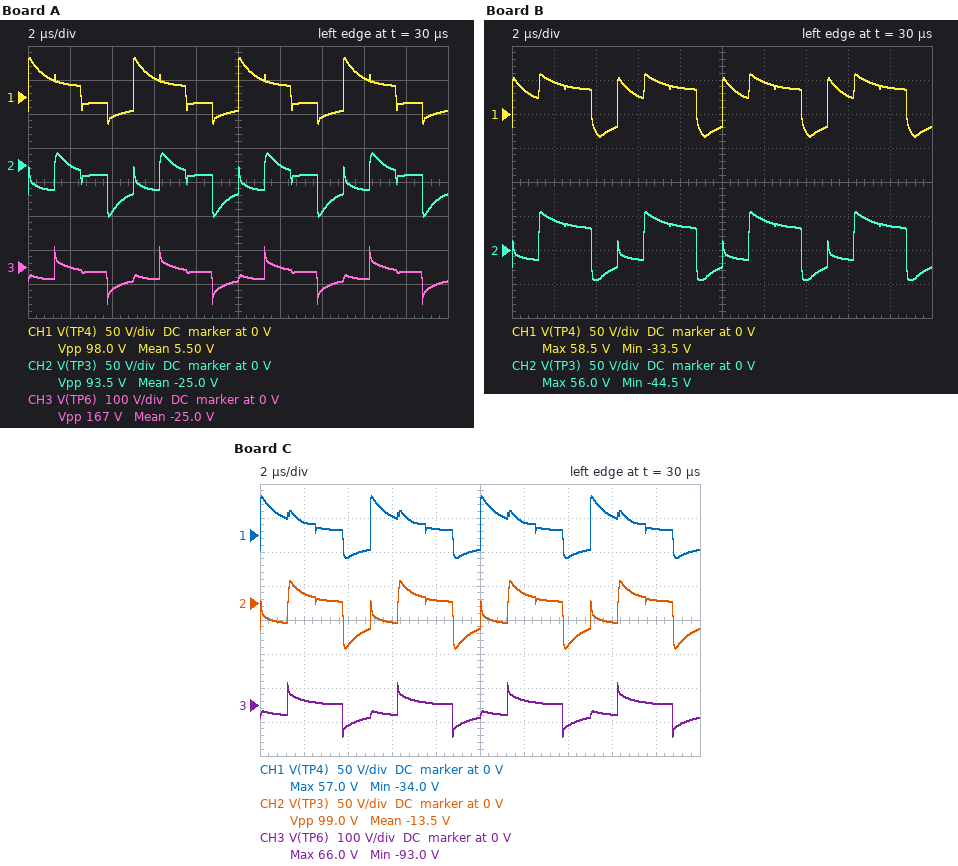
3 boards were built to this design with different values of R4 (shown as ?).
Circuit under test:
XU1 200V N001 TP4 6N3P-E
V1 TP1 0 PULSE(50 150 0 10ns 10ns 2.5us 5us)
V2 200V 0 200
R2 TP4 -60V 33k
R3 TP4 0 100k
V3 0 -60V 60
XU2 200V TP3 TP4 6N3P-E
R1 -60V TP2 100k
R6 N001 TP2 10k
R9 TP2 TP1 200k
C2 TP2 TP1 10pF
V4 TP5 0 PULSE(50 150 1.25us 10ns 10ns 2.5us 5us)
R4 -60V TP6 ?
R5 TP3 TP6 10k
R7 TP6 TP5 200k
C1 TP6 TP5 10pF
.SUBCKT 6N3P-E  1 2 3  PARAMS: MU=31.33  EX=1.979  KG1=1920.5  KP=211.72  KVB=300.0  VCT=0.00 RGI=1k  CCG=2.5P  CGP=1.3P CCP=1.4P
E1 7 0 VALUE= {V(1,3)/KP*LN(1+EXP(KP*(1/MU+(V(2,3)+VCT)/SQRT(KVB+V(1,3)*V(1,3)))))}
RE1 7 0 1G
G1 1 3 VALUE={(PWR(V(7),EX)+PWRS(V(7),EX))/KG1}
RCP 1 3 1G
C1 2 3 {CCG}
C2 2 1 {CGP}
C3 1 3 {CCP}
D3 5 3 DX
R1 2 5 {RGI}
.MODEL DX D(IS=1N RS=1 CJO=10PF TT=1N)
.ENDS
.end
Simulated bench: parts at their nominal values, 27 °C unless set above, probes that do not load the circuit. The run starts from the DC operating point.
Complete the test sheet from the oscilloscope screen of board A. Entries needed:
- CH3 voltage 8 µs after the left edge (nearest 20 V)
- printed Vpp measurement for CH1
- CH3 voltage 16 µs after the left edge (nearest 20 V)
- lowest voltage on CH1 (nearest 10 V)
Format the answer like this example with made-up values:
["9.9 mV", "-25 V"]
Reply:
["-20 V", "98.0 V", "-40 V", "-40 V"]
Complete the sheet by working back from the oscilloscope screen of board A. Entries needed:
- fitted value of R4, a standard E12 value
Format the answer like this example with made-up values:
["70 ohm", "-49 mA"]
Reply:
["56 kΩ"]
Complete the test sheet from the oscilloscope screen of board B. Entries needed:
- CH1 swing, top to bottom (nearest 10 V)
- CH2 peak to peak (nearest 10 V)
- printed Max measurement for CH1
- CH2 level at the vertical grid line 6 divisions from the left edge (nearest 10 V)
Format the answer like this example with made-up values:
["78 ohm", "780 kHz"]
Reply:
["90 V", "100 V", "58.5 V", "40 V"]
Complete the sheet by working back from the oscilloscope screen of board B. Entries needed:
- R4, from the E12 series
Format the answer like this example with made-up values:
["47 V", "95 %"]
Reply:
["150 kΩ"]
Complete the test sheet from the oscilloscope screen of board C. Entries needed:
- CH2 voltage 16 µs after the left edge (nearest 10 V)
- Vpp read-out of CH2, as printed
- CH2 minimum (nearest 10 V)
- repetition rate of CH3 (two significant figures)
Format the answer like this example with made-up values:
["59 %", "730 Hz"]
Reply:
["-30 V", "99.0 V", "-70 V", "200 kHz"]
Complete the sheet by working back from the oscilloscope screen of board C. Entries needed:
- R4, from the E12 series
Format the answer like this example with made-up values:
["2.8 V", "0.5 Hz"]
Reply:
["82 kΩ"]
